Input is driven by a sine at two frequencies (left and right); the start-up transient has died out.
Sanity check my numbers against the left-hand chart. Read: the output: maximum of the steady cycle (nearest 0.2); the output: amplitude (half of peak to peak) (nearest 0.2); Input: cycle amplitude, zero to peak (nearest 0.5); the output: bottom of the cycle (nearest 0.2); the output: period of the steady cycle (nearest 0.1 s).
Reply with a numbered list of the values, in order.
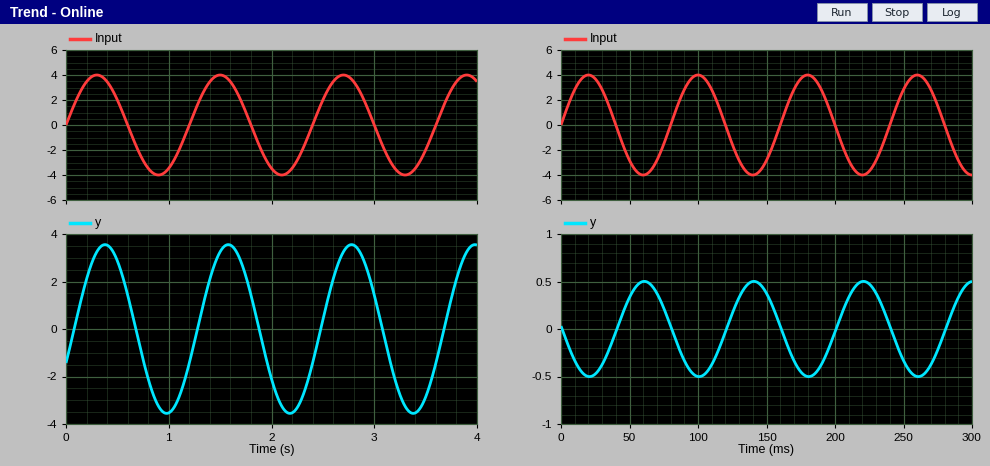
1. 3.6
2. 3.6
3. 4.0
4. -3.6
5. 1.2 s
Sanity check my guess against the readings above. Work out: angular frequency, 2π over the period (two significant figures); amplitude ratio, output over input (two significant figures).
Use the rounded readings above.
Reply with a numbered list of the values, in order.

1. 5.2 rad/s
2. 0.90
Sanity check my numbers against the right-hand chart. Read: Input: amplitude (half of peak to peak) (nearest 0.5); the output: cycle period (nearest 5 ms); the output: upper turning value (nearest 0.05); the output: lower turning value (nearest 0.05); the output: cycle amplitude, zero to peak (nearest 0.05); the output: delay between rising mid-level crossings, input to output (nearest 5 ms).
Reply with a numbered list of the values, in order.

1. 4.0
2. 80 ms
3. 0.50
4. -0.50
5. 0.50
6. 40 ms
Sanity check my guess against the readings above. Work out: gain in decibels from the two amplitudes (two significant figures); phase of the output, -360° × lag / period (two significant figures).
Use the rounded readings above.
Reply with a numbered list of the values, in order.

1. -18 dB
2. -180°
